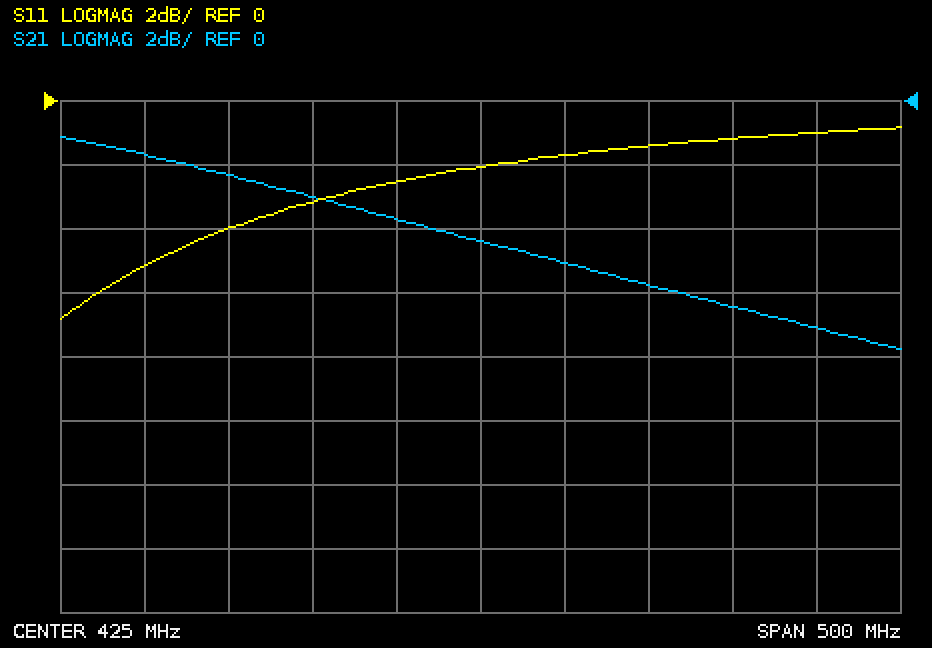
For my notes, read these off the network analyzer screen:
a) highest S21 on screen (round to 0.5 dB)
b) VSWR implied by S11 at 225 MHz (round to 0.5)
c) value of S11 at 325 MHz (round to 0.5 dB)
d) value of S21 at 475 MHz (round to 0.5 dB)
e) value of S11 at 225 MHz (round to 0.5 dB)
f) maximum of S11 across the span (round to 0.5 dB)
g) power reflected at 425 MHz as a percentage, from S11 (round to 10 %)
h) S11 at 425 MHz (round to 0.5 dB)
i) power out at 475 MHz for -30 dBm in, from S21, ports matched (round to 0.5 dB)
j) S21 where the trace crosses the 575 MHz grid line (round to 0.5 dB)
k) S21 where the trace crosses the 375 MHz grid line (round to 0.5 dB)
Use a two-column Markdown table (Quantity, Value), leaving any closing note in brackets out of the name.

| Quantity | Value |
|---|---|
| highest S21 on screen | -1.0 dB |
| VSWR implied by S11 at 225 MHz | 3.5 |
| value of S11 at 325 MHz | -3.0 dB |
| value of S21 at 475 MHz | -5.0 dB |
| value of S11 at 225 MHz | -5.0 dB |
| maximum of S11 across the span | -1.0 dB |
| power reflected at 425 MHz as a percentage, from S11 | 60 % |
| S11 at 425 MHz | -2.0 dB |
| power out at 475 MHz for -30 dBm in, from S21, ports matched | -35.0 dBm |
| S21 where the trace crosses the 575 MHz grid line | -6.5 dB |
| S21 where the trace crosses the 375 MHz grid line | -3.5 dB |
